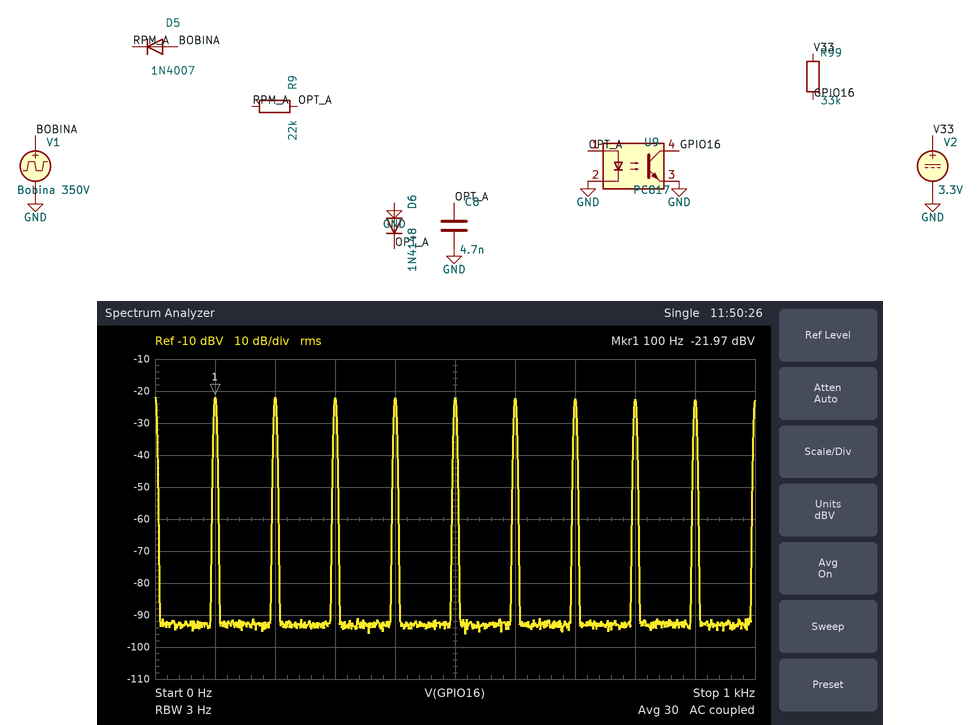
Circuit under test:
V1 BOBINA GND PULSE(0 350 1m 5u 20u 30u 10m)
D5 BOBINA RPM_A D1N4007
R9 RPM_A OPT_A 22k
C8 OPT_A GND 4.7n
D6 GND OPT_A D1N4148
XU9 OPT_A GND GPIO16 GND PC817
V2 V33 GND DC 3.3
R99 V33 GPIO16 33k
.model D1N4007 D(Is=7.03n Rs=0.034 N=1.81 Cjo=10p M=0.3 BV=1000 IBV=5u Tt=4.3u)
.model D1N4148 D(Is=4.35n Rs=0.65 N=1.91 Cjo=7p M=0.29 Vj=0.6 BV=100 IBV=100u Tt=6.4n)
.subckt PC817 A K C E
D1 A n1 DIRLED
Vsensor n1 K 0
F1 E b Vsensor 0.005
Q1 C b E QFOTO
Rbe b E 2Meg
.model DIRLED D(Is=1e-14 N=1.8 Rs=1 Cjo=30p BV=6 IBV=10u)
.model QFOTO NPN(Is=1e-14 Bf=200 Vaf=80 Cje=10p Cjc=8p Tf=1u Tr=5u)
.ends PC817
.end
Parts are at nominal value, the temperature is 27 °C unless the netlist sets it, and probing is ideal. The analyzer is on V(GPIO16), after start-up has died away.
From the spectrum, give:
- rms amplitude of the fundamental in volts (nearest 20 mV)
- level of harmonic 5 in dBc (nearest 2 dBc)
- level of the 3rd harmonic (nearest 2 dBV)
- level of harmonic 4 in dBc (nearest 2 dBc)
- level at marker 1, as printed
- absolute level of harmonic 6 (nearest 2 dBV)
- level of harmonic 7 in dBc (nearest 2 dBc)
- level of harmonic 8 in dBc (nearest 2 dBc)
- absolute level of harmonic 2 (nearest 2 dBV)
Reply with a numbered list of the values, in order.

1. 80 mV
2. 0 dBc
3. -22 dBV
4. 0 dBc
5. -21.97 dBV
6. -22 dBV
7. 0 dBc
8. 0 dBc
9. -22 dBV
